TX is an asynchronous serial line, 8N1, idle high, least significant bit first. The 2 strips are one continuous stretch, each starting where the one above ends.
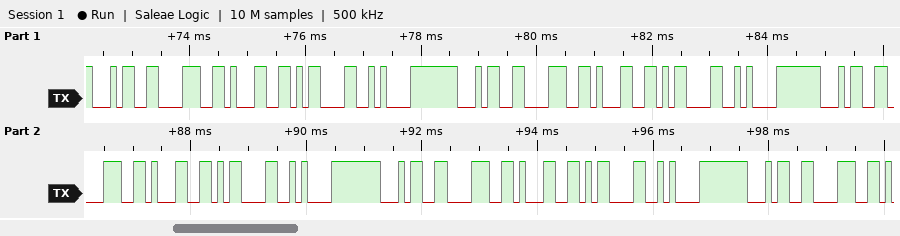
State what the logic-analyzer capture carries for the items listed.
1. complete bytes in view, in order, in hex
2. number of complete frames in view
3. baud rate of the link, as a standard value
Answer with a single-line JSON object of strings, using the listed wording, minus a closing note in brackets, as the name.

{"complete bytes in view, in order, in hex": "34 38 31 0D 0A 34 38 31 0D 0A 34 38 31 0D 0A 34 38 31 0D 0A 34 38", "number of complete frames in view": "22", "baud rate of the link, as a standard value": "9600 baud"}
